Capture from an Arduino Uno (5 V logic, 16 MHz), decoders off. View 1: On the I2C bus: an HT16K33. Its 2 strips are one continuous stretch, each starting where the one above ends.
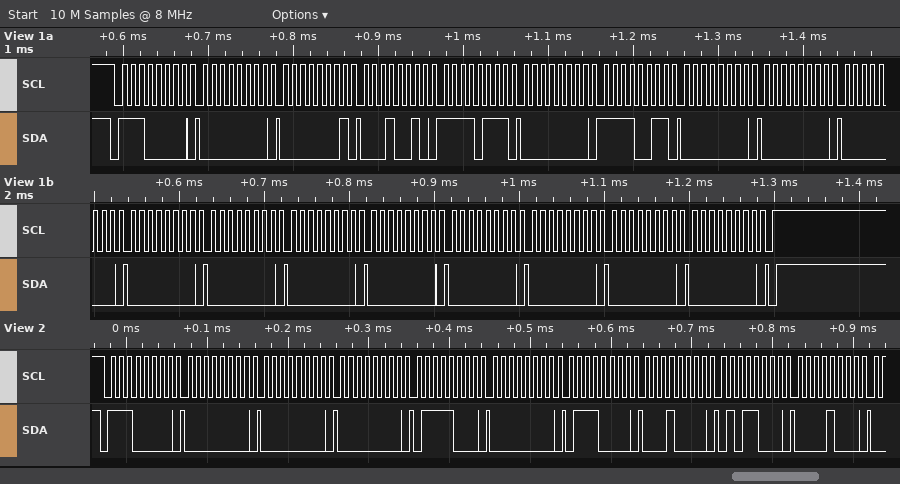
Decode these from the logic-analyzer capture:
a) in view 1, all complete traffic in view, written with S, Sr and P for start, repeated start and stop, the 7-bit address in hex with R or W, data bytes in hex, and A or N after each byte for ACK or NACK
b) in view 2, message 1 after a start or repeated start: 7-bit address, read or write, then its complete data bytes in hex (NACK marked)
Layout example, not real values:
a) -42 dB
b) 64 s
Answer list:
a) S 70W A 00 A 01 A 12 A F7 A 00 A F3 A 00 A 00 A 00 A 00 A 00 A 00 A 00 A 00 A 00 A 00 A 00 A P
b) 0x70 write: 00 00 00 78 00 70 10 58 08
